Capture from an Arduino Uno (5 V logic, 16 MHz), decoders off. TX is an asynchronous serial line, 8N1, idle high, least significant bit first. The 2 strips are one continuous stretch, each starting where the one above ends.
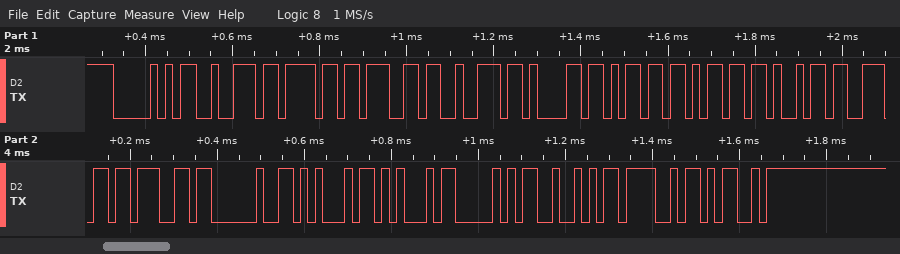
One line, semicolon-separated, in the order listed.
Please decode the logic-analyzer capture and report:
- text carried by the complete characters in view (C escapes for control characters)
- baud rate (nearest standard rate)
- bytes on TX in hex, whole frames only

"Programming EEPROM"; 57600 baud; 50 72 6F 67 72 61 6D 6D 69 6E 67 20 45 45 50 52 4F 4D
